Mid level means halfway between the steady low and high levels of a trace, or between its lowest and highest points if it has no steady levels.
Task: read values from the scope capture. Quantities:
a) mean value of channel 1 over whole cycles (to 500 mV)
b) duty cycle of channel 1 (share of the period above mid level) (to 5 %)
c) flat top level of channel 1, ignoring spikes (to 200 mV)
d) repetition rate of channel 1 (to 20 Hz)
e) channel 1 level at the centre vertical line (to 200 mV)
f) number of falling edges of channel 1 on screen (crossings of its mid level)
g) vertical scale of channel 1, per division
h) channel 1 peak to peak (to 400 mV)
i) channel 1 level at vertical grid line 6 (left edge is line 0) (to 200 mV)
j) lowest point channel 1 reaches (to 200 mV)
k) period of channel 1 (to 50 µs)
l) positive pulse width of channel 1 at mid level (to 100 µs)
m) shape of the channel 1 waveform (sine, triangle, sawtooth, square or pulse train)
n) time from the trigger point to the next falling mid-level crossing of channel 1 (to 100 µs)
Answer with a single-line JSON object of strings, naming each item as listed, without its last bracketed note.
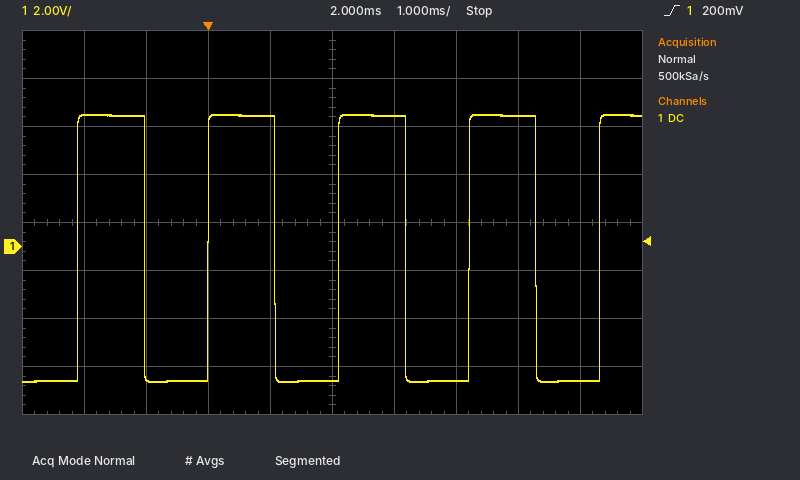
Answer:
{"mean value of channel 1 over whole cycles": "0.0 V", "duty cycle of channel 1 (share of the period above mid level)": "50 %", "flat top level of channel 1, ignoring spikes": "5.4 V", "repetition rate of channel 1": "480 Hz", "channel 1 level at the centre vertical line": "-5.6 V", "number of falling edges of channel 1 on screen": "4", "vertical scale of channel 1, per division": "2 V", "channel 1 peak to peak": "11.2 V", "channel 1 level at vertical grid line 6 (left edge is line 0)": "5.4 V", "lowest point channel 1 reaches": "-5.6 V", "period of channel 1": "2.10 ms", "positive pulse width of channel 1 at mid level": "1.1 ms", "shape of the channel 1 waveform": "square", "time from the trigger point to the next falling mid-level crossing of channel 1": "1.1 ms"}
